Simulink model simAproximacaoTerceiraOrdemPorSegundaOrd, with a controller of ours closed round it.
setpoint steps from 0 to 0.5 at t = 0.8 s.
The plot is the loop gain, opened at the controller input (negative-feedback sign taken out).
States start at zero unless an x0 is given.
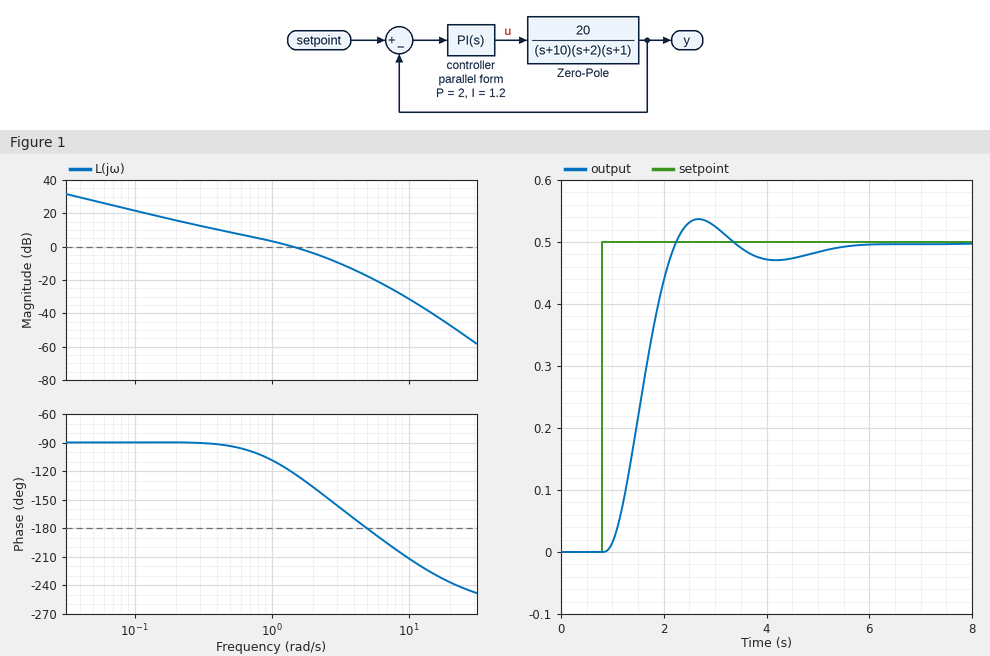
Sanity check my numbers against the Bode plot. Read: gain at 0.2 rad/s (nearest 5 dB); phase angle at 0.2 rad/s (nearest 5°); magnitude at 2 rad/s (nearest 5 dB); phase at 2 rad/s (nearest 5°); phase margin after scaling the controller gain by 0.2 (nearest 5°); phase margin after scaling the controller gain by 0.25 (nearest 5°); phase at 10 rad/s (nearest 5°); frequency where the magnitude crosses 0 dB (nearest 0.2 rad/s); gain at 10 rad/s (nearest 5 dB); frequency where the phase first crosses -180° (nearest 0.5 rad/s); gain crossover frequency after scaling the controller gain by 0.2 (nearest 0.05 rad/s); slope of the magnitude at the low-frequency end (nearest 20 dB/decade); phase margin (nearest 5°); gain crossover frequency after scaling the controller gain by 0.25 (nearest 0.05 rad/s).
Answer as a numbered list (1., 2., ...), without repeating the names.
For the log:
1. 15 dB
2. -90°
3. -5 dB
4. -135°
5. 90°
6. 90°
7. -210°
8. 1.4 rad/s
9. -30 dB
10. 5.0 rad/s
11. 0.25 rad/s
12. -20 dB/decade
13. 60°
14. 0.30 rad/s
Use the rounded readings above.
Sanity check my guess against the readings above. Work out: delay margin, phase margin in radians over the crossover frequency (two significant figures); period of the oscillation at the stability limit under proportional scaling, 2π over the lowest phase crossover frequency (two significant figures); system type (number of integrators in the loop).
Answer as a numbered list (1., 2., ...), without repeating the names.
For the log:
1. 0.75 s
2. 1.3 s
3. 1
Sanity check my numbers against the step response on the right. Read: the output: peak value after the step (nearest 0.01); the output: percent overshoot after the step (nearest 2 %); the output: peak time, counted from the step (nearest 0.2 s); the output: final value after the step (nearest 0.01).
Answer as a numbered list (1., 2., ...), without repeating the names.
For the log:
1. 0.54
2. 8 %
3. 1.8 s
4. 0.50
